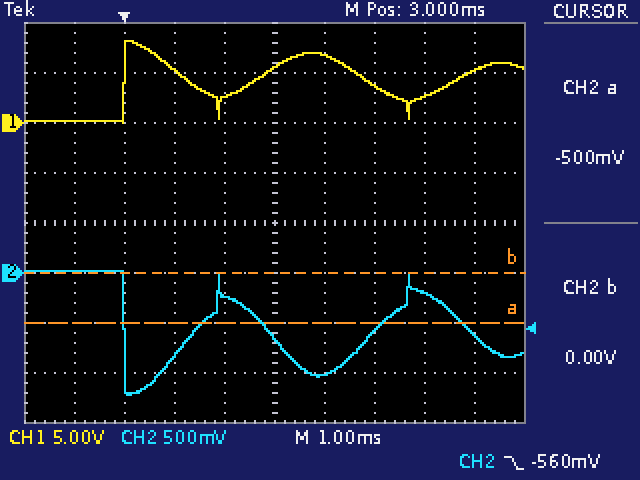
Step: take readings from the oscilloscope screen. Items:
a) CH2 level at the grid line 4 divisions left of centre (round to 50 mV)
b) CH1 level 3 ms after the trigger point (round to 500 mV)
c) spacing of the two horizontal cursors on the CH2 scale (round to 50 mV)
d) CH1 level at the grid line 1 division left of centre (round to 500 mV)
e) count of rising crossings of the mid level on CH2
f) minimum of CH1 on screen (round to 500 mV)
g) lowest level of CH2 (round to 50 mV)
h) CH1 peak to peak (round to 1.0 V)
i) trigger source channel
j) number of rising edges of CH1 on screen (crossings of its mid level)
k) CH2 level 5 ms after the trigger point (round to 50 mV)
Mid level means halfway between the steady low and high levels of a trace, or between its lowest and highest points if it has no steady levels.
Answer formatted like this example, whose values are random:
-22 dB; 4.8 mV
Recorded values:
0 mV; 5.5 V; 500 mV; 2.5 V; 2; 0.0 V; -1.20 V; 8.0 V; CH2; 3; -600 mV
